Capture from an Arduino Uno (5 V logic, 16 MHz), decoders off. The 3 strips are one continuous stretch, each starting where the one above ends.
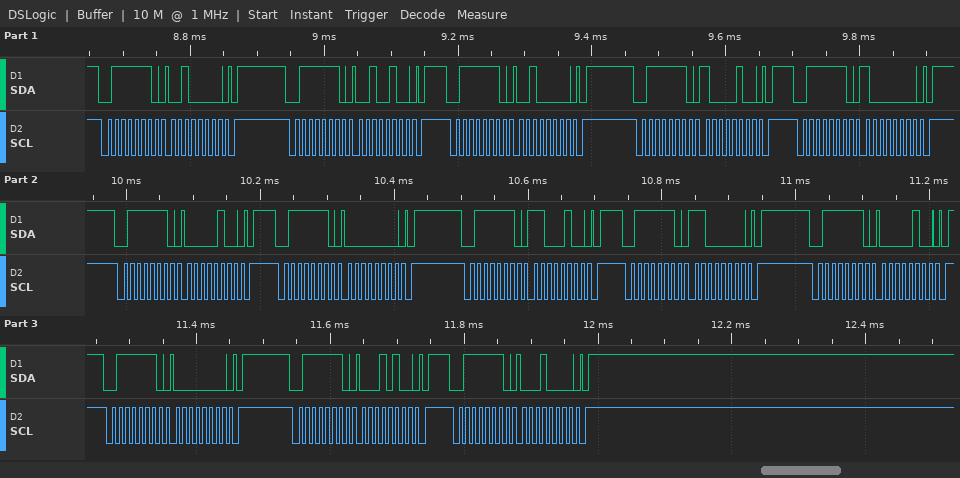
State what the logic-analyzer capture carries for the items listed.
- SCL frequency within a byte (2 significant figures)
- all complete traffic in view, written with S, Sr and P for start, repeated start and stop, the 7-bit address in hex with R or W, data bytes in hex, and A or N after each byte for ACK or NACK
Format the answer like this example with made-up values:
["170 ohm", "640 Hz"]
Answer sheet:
["100 kHz", "S 3FW A 20 A P S 3FW A 24 A P S 3FW A 20 A P S 3FW A 84 A P S 3FW A 80 A P S 3FW A 04 A P S 3FW A 00 A P S 3FW A C4 A P S 3FW A C0 A P S 3FW A 04 A P S 3FW A 00 A P S 3FW A 14 A P S 3FW A 10 A P"]
